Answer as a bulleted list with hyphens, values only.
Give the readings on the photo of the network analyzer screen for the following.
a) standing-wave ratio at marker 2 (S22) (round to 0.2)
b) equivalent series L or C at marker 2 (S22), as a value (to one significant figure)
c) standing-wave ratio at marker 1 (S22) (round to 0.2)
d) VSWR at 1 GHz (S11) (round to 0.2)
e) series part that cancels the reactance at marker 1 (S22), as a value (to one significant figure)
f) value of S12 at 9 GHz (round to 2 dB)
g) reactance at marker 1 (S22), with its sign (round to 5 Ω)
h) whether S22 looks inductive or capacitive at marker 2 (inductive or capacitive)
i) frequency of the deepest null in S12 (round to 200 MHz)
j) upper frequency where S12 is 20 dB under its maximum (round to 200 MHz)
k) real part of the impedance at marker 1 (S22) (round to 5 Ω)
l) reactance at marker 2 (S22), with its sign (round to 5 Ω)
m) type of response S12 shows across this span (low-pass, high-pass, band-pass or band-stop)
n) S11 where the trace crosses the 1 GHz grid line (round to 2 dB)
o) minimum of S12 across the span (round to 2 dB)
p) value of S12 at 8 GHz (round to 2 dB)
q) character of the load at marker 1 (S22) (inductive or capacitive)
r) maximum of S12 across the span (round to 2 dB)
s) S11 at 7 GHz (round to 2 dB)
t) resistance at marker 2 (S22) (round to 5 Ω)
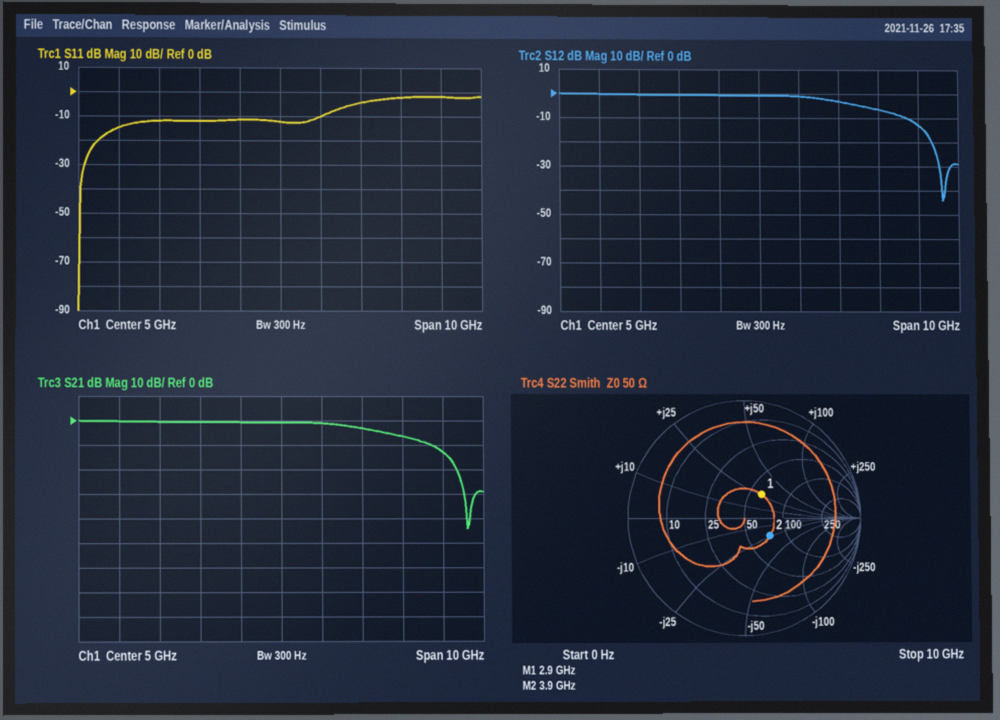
- 1.8
- 2 pF
- 1.6
- 1.4
- 2 pF
- -12 dB
- +25 Ω
- capacitive
- 9.6 GHz
- 9.4 GHz
- 60 Ω
- -25 Ω
- low-pass
- -14 dB
- -44 dB
- -6 dB
- inductive
- 0 dB
- -4 dB
- 75 Ω
